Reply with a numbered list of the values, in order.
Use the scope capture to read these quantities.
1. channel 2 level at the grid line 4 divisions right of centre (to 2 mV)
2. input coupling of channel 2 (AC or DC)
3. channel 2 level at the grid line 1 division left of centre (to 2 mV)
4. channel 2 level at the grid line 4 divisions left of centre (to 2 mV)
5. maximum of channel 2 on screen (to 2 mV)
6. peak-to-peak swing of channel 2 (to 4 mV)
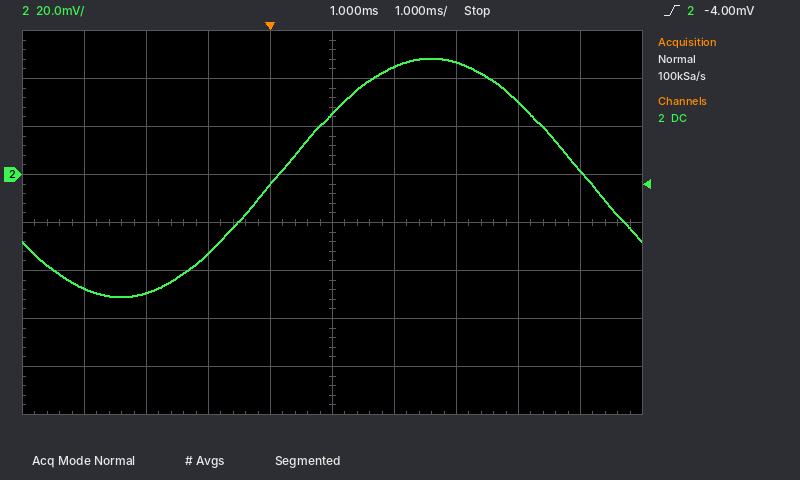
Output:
1. 2 mV
2. DC
3. -4 mV
4. -48 mV
5. 48 mV
6. 100 mV
